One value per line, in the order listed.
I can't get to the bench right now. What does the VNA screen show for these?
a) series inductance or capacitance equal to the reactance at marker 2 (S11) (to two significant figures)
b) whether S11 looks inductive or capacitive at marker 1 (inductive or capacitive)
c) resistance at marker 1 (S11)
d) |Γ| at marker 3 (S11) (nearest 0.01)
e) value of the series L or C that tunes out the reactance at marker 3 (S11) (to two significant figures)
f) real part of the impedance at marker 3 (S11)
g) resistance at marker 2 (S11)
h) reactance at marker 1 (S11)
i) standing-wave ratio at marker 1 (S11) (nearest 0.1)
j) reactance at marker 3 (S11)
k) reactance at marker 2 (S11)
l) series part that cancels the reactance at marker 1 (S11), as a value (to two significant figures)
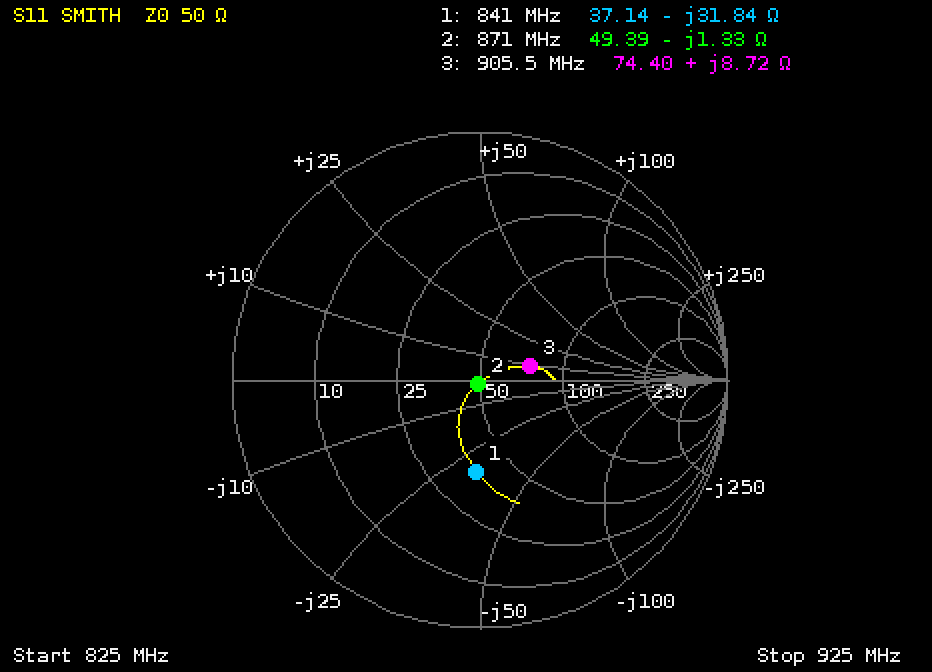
140 pF
capacitive
37.14 Ω
0.21
20 pF
74.40 Ω
49.39 Ω
-31.84 Ω
2.2
+8.72 Ω
-1.33 Ω
6.0 nH
